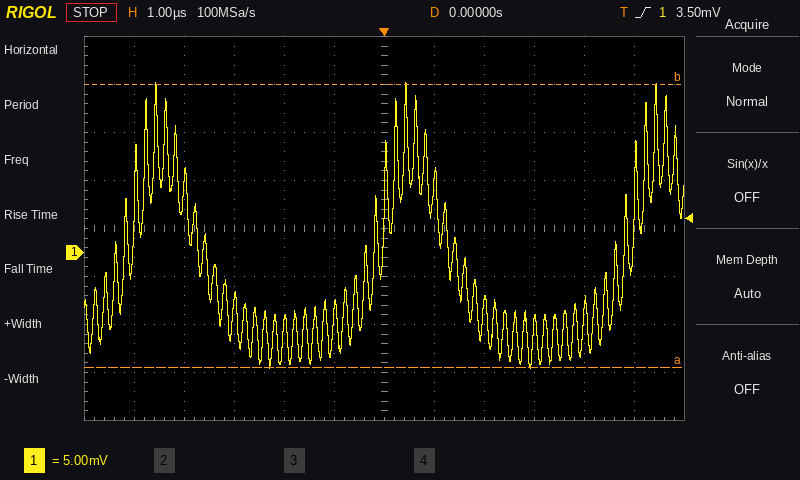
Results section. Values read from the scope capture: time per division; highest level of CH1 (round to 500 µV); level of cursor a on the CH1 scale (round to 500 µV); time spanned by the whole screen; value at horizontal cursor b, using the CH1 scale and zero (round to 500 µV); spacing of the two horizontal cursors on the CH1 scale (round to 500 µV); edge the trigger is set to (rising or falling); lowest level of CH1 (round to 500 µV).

1 µs
17.5 mV
-12.0 mV
12 µs
17.5 mV
29.5 mV
rising
-12.0 mV
